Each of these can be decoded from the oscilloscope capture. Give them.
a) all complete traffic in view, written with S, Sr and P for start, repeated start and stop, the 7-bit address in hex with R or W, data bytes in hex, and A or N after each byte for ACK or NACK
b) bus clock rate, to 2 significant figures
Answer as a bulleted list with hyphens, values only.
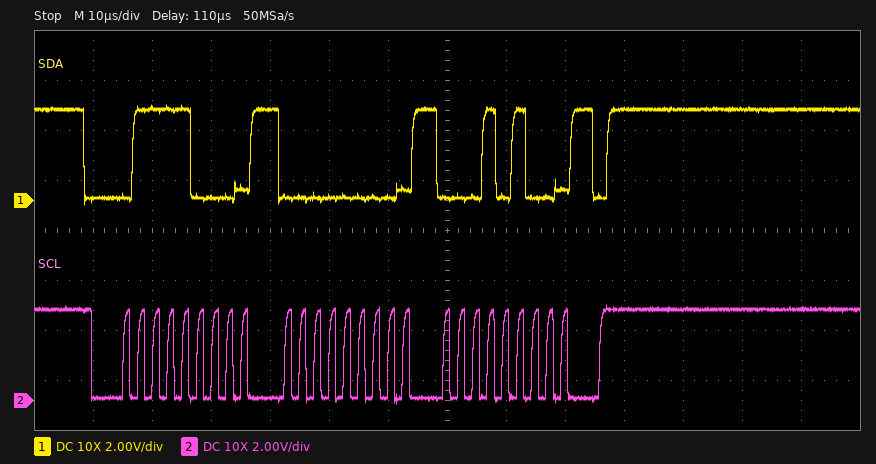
- S 3CW A 00 A 14 A P
- 400 kHz
